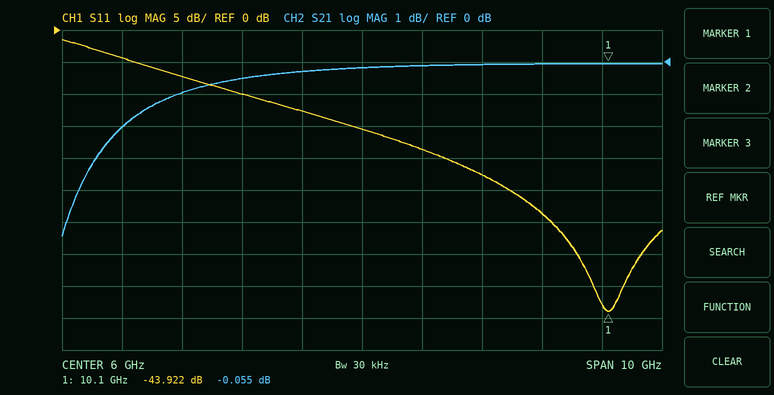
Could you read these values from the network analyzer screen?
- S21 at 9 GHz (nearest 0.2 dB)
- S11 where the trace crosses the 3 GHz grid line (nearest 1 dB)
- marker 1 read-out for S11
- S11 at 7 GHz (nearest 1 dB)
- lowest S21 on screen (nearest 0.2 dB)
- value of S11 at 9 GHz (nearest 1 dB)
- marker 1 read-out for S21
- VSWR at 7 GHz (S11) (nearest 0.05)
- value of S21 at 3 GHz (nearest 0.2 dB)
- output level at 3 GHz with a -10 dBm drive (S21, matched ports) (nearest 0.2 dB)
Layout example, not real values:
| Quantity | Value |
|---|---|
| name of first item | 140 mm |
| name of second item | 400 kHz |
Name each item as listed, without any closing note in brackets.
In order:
| Quantity | Value |
|---|---|
| S21 at 9 GHz | 0.0 dB |
| S11 where the trace crosses the 3 GHz grid line | -7 dB |
| marker 1 read-out for S11 | -43.922 dB |
| S11 at 7 GHz | -19 dB |
| lowest S21 on screen | -5.4 dB |
| value of S11 at 9 GHz | -29 dB |
| marker 1 read-out for S21 | -0.055 dB |
| VSWR at 7 GHz (S11) | 1.25 |
| value of S21 at 3 GHz | -1.0 dB |
| output level at 3 GHz with a -10 dBm drive (S21, matched ports) | -11.0 dBm |
